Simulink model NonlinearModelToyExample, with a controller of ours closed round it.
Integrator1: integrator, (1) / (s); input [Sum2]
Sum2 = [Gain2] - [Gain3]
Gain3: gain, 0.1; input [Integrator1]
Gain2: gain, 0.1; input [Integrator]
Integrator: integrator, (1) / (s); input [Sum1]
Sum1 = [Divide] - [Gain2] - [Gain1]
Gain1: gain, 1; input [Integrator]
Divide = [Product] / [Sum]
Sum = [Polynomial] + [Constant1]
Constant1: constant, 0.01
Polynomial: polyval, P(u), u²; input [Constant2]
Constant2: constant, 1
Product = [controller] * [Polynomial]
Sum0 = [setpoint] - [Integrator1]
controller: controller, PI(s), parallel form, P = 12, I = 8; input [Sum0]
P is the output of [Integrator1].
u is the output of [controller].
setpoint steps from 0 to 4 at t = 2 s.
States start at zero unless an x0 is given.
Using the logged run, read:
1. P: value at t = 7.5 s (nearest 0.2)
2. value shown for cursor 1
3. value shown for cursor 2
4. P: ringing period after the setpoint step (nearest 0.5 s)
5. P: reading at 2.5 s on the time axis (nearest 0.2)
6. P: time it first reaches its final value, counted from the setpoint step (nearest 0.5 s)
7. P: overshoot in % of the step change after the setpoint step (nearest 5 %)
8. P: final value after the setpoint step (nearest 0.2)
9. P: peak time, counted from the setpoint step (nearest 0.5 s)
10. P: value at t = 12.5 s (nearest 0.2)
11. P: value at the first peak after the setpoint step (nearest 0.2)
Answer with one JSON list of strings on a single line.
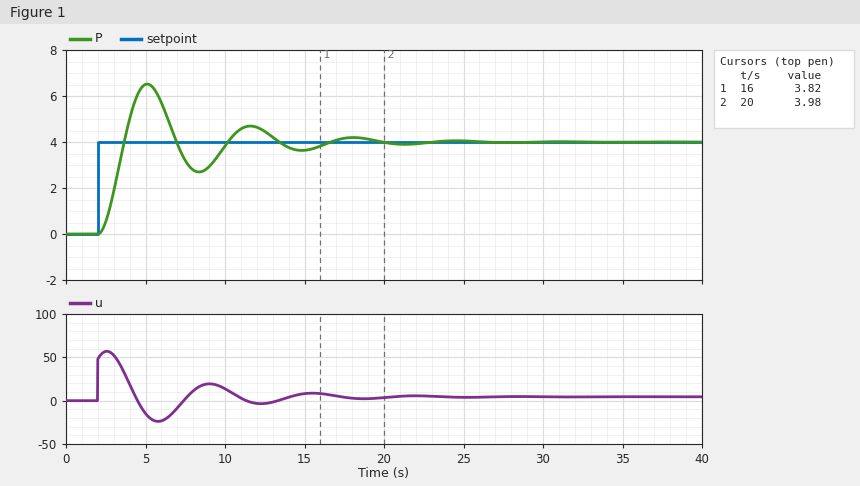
["3.2", "3.82", "3.98", "6.5 s", "0.6", "1.5 s", "65 %", "4.0", "3.0 s", "4.4", "6.6"]
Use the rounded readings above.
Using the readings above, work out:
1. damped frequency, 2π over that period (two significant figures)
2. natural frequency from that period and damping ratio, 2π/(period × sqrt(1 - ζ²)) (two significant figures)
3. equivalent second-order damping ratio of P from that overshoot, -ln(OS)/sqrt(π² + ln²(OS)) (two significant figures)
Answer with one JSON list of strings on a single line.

["0.97 rad/s", "0.98 rad/s", "0.14"]
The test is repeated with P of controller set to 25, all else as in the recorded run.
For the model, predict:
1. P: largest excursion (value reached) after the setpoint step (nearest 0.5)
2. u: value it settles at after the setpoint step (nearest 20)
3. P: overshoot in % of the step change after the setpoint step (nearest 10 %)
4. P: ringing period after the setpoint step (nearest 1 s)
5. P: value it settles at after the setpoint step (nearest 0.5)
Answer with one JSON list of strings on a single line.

["6.0", "0", "50 %", "4 s", "4.0"]
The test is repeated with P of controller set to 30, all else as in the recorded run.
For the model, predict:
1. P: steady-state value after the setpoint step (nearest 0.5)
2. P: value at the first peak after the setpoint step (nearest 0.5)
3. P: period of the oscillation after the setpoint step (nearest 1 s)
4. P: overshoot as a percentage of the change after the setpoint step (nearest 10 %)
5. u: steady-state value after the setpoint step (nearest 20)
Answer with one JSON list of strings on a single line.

["4.0", "6.0", "4 s", "50 %", "0"]
